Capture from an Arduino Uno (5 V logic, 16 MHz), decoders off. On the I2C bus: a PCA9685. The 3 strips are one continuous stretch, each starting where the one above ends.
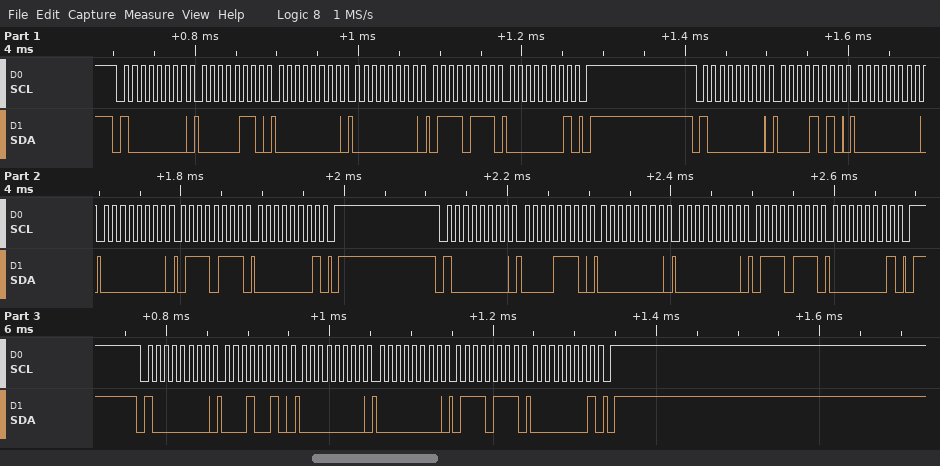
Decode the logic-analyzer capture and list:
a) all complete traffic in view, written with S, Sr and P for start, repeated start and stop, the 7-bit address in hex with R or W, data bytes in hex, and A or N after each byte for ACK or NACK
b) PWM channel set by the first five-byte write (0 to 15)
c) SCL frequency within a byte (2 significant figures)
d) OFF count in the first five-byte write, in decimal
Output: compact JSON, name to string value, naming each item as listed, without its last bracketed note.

{"all complete traffic in view, written with S, Sr and P for start, repeated start and stop, the 7-bit address in hex with R or W, data bytes in hex, and A or N after each byte for ACK or NACK": "S 40W A 06 A 00 A 00 A 77 A 01 A P S 40W A 0A A 00 A 00 A 77 A 01 A P S 40W A 0E A 00 A 00 A 77 A 01 A P S 40W A 12 A 00 A 00 A 77 A 01 A P", "PWM channel set by the first five-byte write": "0", "SCL frequency within a byte": "100 kHz", "OFF count in the first five-byte write, in decimal": "375"}
